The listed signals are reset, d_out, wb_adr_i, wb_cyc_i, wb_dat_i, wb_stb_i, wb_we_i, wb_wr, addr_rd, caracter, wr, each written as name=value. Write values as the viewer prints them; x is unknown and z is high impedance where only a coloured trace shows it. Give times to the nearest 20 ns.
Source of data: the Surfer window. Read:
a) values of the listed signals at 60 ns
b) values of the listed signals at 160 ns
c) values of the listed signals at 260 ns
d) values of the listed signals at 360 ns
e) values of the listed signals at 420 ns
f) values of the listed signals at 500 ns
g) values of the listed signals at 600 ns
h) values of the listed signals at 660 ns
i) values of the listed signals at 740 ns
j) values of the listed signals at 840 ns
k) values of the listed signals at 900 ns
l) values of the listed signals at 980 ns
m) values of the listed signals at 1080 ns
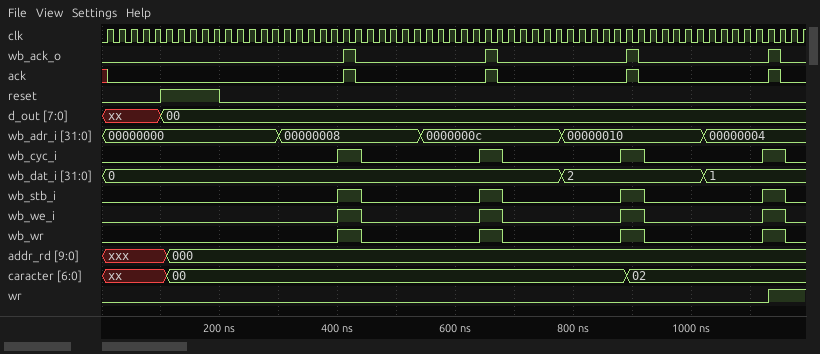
reset=0, d_out=xx, wb_adr_i=00000000, wb_cyc_i=0, wb_dat_i=0, wb_stb_i=0, wb_we_i=0, wb_wr=0, addr_rd=xxx, caracter=xx, wr=0
reset=1, d_out=00, wb_adr_i=00000000, wb_cyc_i=0, wb_dat_i=0, wb_stb_i=0, wb_we_i=0, wb_wr=0, addr_rd=000, caracter=00, wr=0
reset=0, d_out=00, wb_adr_i=00000000, wb_cyc_i=0, wb_dat_i=0, wb_stb_i=0, wb_we_i=0, wb_wr=0, addr_rd=000, caracter=00, wr=0
reset=0, d_out=00, wb_adr_i=00000008, wb_cyc_i=0, wb_dat_i=0, wb_stb_i=0, wb_we_i=0, wb_wr=0, addr_rd=000, caracter=00, wr=0
reset=0, d_out=00, wb_adr_i=00000008, wb_cyc_i=1, wb_dat_i=0, wb_stb_i=1, wb_we_i=1, wb_wr=1, addr_rd=000, caracter=00, wr=0
reset=0, d_out=00, wb_adr_i=00000008, wb_cyc_i=0, wb_dat_i=0, wb_stb_i=0, wb_we_i=0, wb_wr=0, addr_rd=000, caracter=00, wr=0
reset=0, d_out=00, wb_adr_i=0000000c, wb_cyc_i=0, wb_dat_i=0, wb_stb_i=0, wb_we_i=0, wb_wr=0, addr_rd=000, caracter=00, wr=0
reset=0, d_out=00, wb_adr_i=0000000c, wb_cyc_i=1, wb_dat_i=0, wb_stb_i=1, wb_we_i=1, wb_wr=1, addr_rd=000, caracter=00, wr=0
reset=0, d_out=00, wb_adr_i=0000000c, wb_cyc_i=0, wb_dat_i=0, wb_stb_i=0, wb_we_i=0, wb_wr=0, addr_rd=000, caracter=00, wr=0
reset=0, d_out=00, wb_adr_i=00000010, wb_cyc_i=0, wb_dat_i=2, wb_stb_i=0, wb_we_i=0, wb_wr=0, addr_rd=000, caracter=00, wr=0
reset=0, d_out=00, wb_adr_i=00000010, wb_cyc_i=1, wb_dat_i=2, wb_stb_i=1, wb_we_i=1, wb_wr=1, addr_rd=000, caracter=02, wr=0
reset=0, d_out=00, wb_adr_i=00000010, wb_cyc_i=0, wb_dat_i=2, wb_stb_i=0, wb_we_i=0, wb_wr=0, addr_rd=000, caracter=02, wr=0
reset=0, d_out=00, wb_adr_i=00000004, wb_cyc_i=0, wb_dat_i=1, wb_stb_i=0, wb_we_i=0, wb_wr=0, addr_rd=000, caracter=02, wr=0
